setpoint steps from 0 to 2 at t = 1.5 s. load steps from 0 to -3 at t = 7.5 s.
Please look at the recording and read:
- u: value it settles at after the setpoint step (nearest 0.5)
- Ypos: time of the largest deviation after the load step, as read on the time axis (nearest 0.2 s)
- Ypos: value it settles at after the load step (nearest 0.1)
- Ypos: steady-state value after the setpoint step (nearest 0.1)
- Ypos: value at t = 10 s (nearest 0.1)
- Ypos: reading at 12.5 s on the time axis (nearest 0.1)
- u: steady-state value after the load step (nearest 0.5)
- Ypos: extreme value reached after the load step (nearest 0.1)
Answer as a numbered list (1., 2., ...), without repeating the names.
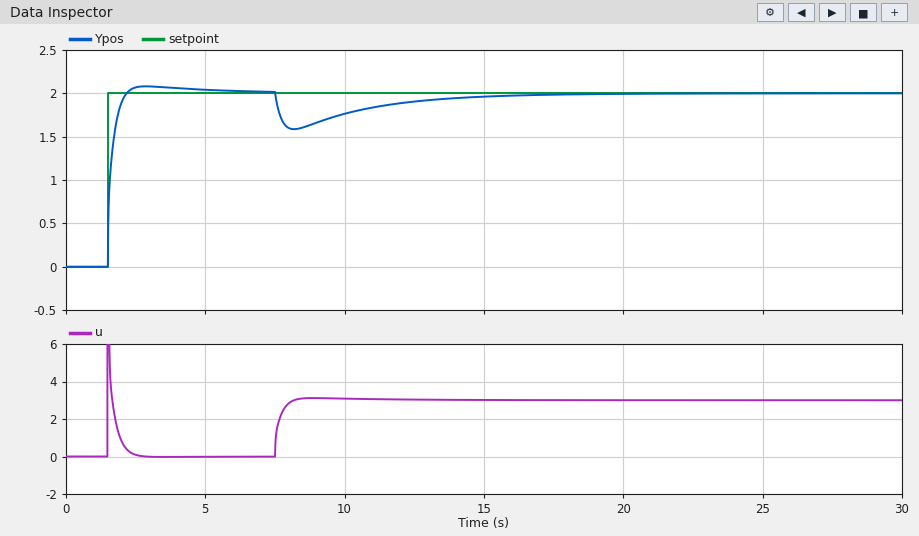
1. 0.0
2. 8.2 s
3. 2.0
4. 2.0
5. 1.8
6. 1.9
7. 3.0
8. 1.6
